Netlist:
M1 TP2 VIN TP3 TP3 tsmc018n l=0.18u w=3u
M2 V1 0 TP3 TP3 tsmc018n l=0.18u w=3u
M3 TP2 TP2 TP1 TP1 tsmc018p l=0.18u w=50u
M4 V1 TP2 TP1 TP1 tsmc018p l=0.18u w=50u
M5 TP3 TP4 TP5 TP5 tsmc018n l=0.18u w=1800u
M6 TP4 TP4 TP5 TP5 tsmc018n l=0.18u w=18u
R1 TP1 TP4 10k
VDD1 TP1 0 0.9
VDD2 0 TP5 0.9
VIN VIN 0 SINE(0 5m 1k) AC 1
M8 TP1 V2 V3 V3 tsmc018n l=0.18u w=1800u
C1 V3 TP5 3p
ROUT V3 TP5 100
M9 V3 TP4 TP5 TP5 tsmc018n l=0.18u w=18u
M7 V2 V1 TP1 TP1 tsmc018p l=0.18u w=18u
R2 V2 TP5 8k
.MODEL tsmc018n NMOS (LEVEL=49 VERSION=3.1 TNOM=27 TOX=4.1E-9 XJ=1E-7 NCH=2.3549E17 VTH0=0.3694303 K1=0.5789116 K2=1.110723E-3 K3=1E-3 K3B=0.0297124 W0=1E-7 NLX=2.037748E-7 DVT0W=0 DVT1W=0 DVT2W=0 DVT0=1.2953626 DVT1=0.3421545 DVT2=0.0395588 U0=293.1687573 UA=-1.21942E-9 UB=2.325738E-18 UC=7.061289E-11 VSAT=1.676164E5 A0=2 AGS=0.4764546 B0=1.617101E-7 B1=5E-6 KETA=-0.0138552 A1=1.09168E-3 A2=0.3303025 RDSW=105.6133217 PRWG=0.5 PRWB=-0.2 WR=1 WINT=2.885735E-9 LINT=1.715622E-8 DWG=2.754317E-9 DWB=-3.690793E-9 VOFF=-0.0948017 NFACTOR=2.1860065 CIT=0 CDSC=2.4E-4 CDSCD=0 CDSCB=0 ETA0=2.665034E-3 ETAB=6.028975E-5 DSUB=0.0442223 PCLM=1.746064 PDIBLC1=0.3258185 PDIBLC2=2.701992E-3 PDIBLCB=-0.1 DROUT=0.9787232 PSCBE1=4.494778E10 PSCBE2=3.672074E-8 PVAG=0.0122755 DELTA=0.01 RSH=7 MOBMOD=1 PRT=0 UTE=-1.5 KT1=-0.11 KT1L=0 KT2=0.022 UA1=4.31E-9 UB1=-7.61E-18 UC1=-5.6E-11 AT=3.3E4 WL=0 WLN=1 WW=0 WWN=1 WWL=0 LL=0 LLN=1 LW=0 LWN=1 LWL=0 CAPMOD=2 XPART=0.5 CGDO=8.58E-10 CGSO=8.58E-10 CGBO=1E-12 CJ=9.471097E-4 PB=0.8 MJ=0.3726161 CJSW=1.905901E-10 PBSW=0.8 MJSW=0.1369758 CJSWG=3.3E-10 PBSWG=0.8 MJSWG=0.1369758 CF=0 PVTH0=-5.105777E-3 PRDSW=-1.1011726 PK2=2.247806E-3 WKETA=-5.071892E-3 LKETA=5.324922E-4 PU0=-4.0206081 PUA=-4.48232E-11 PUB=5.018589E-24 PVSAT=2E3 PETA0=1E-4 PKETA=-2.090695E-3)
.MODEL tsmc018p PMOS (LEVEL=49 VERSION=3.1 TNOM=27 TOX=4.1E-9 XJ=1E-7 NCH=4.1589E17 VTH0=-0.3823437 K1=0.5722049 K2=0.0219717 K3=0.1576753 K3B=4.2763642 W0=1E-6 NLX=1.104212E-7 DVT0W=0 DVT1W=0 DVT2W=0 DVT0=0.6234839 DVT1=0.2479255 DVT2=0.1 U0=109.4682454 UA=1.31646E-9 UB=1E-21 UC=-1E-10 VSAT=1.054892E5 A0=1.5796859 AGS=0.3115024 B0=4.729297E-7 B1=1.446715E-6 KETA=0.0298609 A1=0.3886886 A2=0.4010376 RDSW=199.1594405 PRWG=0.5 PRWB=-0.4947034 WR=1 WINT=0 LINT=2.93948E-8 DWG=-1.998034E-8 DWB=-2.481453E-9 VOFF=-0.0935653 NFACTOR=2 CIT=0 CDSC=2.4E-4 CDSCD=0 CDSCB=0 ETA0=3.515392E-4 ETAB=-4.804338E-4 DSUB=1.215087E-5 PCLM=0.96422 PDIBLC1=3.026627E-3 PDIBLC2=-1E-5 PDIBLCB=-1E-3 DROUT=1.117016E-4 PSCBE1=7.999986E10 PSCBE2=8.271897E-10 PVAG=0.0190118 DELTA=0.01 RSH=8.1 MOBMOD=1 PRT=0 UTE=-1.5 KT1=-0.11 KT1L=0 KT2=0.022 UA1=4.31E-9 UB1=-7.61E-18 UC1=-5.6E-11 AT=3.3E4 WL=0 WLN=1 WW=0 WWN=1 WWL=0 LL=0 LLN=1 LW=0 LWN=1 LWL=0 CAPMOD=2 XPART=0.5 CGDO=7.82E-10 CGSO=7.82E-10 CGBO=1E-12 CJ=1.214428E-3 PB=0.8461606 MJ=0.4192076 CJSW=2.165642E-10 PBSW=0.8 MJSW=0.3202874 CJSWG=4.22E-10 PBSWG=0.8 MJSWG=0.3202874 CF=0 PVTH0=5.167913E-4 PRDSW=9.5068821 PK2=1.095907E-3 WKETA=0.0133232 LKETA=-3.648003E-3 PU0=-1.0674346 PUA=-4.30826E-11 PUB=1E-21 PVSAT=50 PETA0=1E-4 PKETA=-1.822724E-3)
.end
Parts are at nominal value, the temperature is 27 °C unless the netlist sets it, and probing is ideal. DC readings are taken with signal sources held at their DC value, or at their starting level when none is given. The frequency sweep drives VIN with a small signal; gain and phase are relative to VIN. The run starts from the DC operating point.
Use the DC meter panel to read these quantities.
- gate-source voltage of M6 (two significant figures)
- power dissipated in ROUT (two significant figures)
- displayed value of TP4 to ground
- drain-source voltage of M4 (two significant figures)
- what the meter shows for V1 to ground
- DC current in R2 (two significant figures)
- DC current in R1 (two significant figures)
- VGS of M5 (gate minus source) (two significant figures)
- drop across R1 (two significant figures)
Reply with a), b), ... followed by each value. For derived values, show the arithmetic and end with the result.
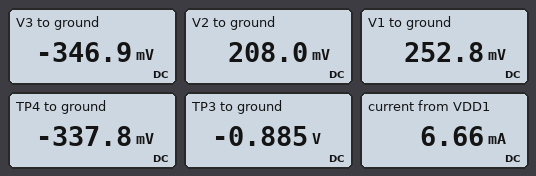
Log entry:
a) -337.8 mV - (-900 mV) = 560 mV
b) (-346.9 mV - (-900 mV))^2 / 100 Ω = 3.1 mW
c) -337.8 mV
d) 252.8 mV - 900 mV = -650 mV
e) 252.8 mV
f) (208 mV - (-900 mV)) / 8 kΩ = 140 µA
g) (900 mV - (-337.8 mV)) / 10 kΩ = 120 µA
h) -337.8 mV - (-900 mV) = 560 mV
i) 900 mV - (-337.8 mV) = 1.2 V
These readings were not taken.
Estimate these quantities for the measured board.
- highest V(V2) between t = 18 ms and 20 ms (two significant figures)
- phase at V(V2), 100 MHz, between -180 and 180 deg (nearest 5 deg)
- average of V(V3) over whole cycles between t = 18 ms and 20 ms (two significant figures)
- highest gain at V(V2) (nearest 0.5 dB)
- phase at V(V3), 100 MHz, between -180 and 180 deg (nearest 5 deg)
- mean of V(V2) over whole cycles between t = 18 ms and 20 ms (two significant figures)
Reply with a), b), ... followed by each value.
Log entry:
a) 690 mV
b) 55 deg
c) -340 mV
d) 41.5 dB
e) 55 deg
f) 210 mV
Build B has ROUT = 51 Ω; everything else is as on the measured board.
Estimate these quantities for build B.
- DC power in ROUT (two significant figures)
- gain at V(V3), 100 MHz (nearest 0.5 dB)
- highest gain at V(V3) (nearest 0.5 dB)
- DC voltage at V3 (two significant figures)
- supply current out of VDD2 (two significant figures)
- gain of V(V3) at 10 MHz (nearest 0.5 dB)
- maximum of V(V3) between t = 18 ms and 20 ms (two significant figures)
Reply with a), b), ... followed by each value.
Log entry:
a) 4.7 mW
b) 17.0 dB
c) 39.0 dB
d) -410 mV
e) 11 mA
f) 36.0 dB
g) -34 mV
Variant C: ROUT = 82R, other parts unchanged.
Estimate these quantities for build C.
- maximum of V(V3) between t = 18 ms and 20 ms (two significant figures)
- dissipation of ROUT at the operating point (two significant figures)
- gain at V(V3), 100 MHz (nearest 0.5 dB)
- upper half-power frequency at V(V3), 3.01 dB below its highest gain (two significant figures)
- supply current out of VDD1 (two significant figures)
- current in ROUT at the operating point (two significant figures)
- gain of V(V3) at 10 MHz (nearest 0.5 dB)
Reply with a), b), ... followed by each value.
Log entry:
a) 37 mV
b) 3.5 mW
c) 18.0 dB
d) 10 MHz
e) 7.7 mA
f) 6.5 mA
g) 36.5 dB
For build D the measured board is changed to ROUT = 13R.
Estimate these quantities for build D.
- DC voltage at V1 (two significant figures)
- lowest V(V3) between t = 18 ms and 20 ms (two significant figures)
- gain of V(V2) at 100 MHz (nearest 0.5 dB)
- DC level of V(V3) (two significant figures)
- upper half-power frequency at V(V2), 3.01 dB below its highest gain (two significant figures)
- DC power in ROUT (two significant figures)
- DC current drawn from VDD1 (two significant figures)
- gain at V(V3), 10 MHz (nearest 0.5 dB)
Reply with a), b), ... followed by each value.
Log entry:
a) 250 mV
b) -840 mV
c) 17.5 dB
d) -590 mV
e) 8.0 MHz
f) 7.5 mW
g) 25 mA
h) 31.5 dB
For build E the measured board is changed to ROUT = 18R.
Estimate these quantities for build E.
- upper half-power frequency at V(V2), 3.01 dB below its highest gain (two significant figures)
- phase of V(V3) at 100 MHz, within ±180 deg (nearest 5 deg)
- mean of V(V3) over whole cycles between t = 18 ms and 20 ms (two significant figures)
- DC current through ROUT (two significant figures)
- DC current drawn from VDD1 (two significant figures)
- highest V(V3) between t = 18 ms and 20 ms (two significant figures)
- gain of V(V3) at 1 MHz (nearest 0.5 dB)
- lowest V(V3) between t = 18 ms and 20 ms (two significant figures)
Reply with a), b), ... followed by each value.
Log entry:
a) 8.4 MHz
b) 55 deg
c) -540 mV
d) 20 mA
e) 21 mA
f) -250 mV
g) 36.5 dB
h) -820 mV
